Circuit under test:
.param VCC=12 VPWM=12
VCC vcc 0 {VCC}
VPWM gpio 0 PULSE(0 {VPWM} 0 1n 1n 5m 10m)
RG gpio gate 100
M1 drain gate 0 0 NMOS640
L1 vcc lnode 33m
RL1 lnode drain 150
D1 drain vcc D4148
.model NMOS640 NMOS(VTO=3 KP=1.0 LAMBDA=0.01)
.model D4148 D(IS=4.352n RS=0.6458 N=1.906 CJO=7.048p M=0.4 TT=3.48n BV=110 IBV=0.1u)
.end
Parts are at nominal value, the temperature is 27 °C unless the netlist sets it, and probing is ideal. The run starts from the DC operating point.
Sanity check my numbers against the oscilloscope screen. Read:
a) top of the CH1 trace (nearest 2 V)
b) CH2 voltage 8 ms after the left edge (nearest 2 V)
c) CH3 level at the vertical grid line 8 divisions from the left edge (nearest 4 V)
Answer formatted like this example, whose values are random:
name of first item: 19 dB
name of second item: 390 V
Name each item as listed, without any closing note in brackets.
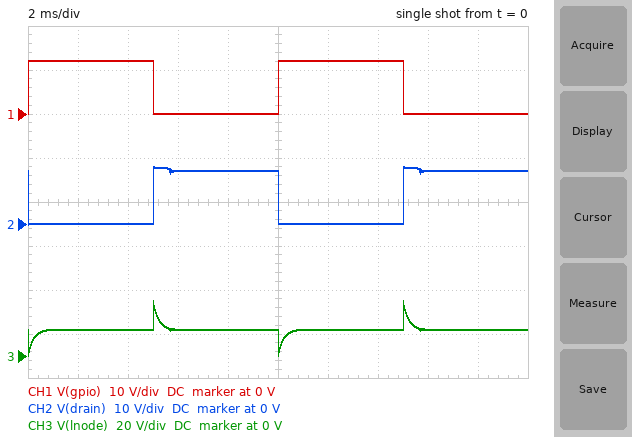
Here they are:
top of the CH1 trace: 12 V
CH2 voltage 8 ms after the left edge: 12 V
CH3 level at the vertical grid line 8 divisions from the left edge: 12 V
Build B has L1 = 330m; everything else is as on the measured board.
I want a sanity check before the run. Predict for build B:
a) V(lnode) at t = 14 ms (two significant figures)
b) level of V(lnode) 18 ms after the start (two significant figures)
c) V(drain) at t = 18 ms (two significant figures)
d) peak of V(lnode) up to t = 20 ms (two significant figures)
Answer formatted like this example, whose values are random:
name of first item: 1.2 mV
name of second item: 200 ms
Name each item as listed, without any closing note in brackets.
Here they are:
V(lnode) at t = 14 ms: 10 V
level of V(lnode) 18 ms after the start: 15 V
V(drain) at t = 18 ms: 13 V
peak of V(lnode) up to t = 20 ms: 24 V
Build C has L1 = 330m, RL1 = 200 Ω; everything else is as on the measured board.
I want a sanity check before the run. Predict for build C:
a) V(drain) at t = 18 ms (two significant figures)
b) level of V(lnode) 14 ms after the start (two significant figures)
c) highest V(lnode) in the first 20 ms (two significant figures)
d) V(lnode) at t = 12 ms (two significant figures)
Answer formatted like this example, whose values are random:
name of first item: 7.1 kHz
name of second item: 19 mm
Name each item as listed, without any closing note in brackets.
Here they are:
V(drain) at t = 18 ms: 13 V
level of V(lnode) 14 ms after the start: 11 V
highest V(lnode) in the first 20 ms: 24 V
V(lnode) at t = 12 ms: 8.4 V
